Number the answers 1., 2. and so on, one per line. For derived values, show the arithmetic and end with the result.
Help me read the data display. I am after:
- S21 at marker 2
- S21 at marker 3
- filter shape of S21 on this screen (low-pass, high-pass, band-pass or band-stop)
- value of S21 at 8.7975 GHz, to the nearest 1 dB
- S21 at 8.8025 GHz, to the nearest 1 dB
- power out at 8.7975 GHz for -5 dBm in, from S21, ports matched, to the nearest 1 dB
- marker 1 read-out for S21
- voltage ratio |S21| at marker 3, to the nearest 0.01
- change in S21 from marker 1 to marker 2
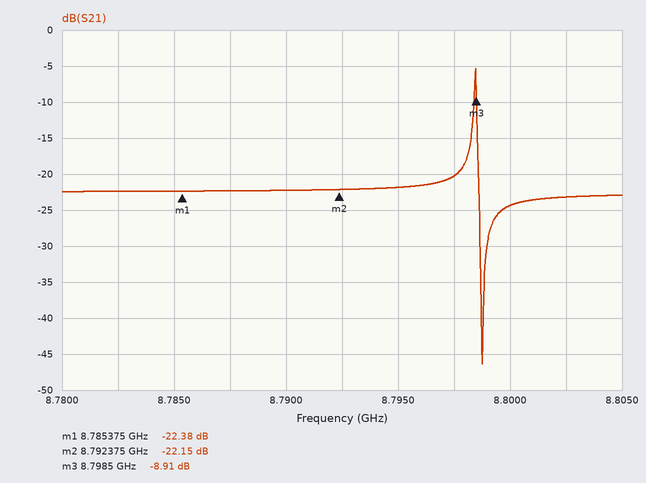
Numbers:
1. -22.15 dB
2. -8.91 dB
3. band-pass
4. -20 dB
5. -23 dB
6. -5 dBm + (-20 dB) = -25 dBm
7. -22.38 dB
8. 10^(-8.91/20) ≈ 0.36
9. -22.15 − (-22.38) = 0.23 dB
